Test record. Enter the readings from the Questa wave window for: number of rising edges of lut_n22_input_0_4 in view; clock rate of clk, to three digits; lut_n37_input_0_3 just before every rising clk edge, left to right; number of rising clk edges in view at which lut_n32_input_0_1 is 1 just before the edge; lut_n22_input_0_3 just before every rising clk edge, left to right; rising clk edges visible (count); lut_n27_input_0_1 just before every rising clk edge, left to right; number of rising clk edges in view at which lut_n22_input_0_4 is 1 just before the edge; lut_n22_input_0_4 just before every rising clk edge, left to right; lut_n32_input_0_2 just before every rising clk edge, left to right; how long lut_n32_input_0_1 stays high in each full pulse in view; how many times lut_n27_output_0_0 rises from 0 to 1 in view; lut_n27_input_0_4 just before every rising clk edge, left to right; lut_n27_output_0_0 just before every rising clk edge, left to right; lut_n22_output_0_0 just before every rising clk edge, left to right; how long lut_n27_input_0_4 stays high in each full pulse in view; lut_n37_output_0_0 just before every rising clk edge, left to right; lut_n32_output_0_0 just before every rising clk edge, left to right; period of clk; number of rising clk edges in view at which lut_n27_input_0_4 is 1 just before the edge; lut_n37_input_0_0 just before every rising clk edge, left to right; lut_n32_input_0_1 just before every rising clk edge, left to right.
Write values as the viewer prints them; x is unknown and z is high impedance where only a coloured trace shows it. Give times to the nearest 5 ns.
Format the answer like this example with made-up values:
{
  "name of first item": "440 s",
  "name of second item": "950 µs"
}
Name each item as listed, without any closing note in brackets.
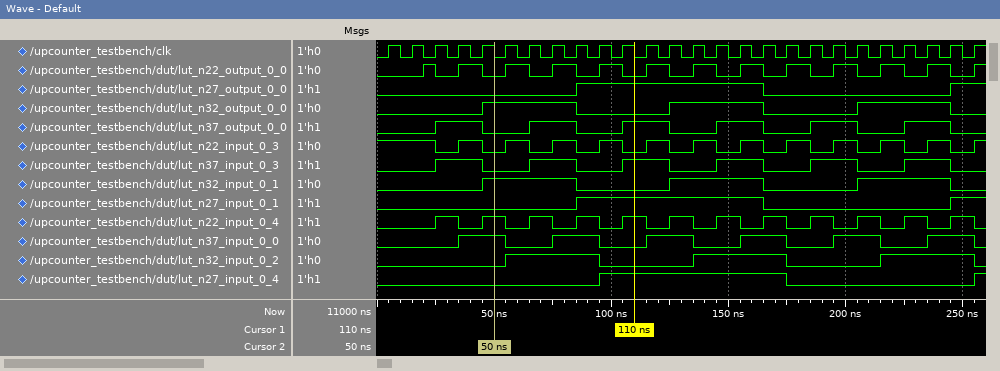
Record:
{
  "number of rising edges of lut_n22_input_0_4 in view": "12",
  "clock rate of clk, to three digits": "100 MHz",
  "lut_n37_input_0_3 just before every rising clk edge, left to right": "0 0 0 1 1 0 0 1 1 0 0 1 1 0 0 1 1 0 0 1 1 0 0 1 1 0",
  "number of rising clk edges in view at which lut_n32_input_0_1 is 1 just before the edge": "12",
  "lut_n22_input_0_3 just before every rising clk edge, left to right": "1 1 1 0 1 0 1 0 1 0 1 0 1 0 1 0 1 0 1 0 1 0 1 0 1 0",
  "rising clk edges visible": "26",
  "lut_n27_input_0_1 just before every rising clk edge, left to right": "0 0 0 0 0 0 0 0 0 1 1 1 1 1 1 1 1 0 0 0 0 0 0 0 0 1",
  "number of rising clk edges in view at which lut_n22_input_0_4 is 1 just before the edge": "12",
  "lut_n22_input_0_4 just before every rising clk edge, left to right": "0 0 0 1 0 1 0 1 0 1 0 1 0 1 0 1 0 1 0 1 0 1 0 1 0 1",
  "lut_n32_input_0_2 just before every rising clk edge, left to right": "0 0 0 0 0 0 1 1 1 1 0 0 0 0 1 1 1 1 0 0 0 0 1 1 1 1",
  "how long lut_n32_input_0_1 stays high in each full pulse in view": "40 ns, 40 ns, 40 ns",
  "how many times lut_n27_output_0_0 rises from 0 to 1 in view": "2",
  "lut_n27_input_0_4 just before every rising clk edge, left to right": "0 0 0 0 0 0 0 0 0 0 1 1 1 1 1 1 1 1 0 0 0 0 0 0 0 0",
  "lut_n27_output_0_0 just before every rising clk edge, left to right": "0 0 0 0 0 0 0 0 0 1 1 1 1 1 1 1 1 0 0 0 0 0 0 0 0 1",
  "lut_n22_output_0_0 just before every rising clk edge, left to right": "0 0 1 0 1 0 1 0 1 0 1 0 1 0 1 0 1 0 1 0 1 0 1 0 1 0",
  "how long lut_n27_input_0_4 stays high in each full pulse in view": "80 ns",
  "lut_n37_output_0_0 just before every rising clk edge, left to right": "0 0 0 1 1 0 0 1 1 0 0 1 1 0 0 1 1 0 0 1 1 0 0 1 1 0",
  "lut_n32_output_0_0 just before every rising clk edge, left to right": "0 0 0 0 0 1 1 1 1 0 0 0 0 1 1 1 1 0 0 0 0 1 1 1 1 0",
  "period of clk": "10 ns",
  "number of rising clk edges in view at which lut_n27_input_0_4 is 1 just before the edge": "8",
  "lut_n37_input_0_0 just before every rising clk edge, left to right": "0 0 0 0 1 1 0 0 1 1 0 0 1 1 0 0 1 1 0 0 1 1 0 0 1 1",
  "lut_n32_input_0_1 just before every rising clk edge, left to right": "0 0 0 0 0 1 1 1 1 0 0 0 0 1 1 1 1 0 0 0 0 1 1 1 1 0"
}
